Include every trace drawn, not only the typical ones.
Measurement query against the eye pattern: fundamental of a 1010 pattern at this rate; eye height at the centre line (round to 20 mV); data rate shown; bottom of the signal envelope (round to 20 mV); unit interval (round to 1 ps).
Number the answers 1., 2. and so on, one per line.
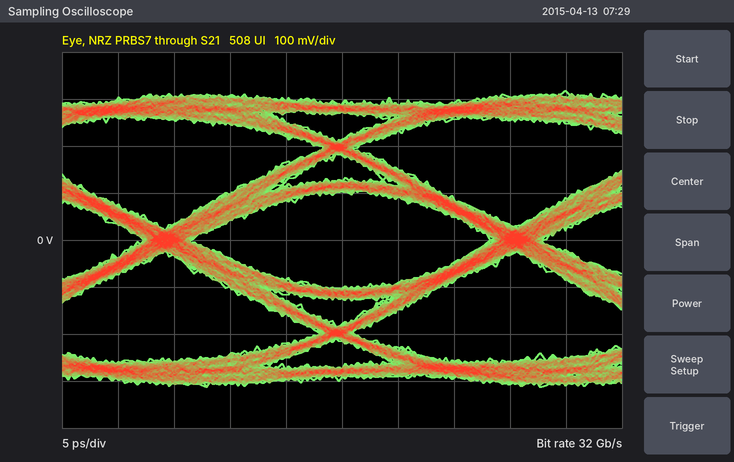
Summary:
1. 16 GHz
2. 200 mV
3. 32 Gb/s
4. -320 mV
5. 31 ps
